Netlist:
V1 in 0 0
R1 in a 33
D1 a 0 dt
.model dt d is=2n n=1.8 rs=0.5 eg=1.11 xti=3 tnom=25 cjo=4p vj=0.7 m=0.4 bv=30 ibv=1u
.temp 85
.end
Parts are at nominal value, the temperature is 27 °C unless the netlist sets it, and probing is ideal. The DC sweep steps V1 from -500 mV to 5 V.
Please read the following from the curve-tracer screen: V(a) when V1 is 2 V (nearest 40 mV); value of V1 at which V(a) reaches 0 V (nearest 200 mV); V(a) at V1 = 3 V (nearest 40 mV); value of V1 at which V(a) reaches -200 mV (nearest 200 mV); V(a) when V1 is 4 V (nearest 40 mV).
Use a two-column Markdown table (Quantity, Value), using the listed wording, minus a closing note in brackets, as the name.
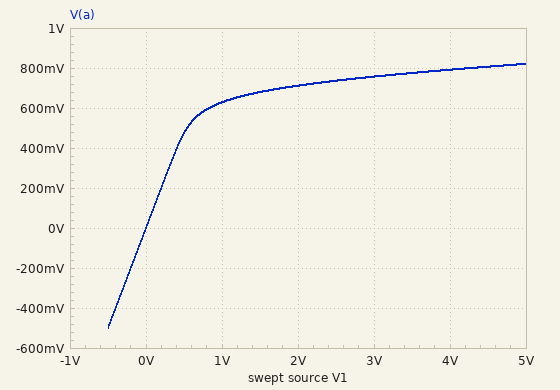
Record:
| Quantity | Value |
|---|---|
| V(a) when V1 is 2 V | 720 mV |
| value of V1 at which V(a) reaches 0 V | 0 V |
| V(a) at V1 = 3 V | 760 mV |
| value of V1 at which V(a) reaches -200 mV | -200 mV |
| V(a) when V1 is 4 V | 800 mV |
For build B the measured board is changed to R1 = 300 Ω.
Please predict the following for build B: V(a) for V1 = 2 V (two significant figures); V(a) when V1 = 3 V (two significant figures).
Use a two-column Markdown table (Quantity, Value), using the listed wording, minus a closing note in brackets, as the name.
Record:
| Quantity | Value |
|---|---|
| V(a) for V1 = 2 V | 580 mV |
| V(a) when V1 = 3 V | 610 mV |
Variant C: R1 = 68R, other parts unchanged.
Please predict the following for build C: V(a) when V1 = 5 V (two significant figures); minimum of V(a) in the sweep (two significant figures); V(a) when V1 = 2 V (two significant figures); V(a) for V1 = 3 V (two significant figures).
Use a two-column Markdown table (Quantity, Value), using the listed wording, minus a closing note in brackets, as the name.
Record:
| Quantity | Value |
|---|---|
| V(a) when V1 = 5 V | 750 mV |
| minimum of V(a) in the sweep | -500 mV |
| V(a) when V1 = 2 V | 660 mV |
| V(a) for V1 = 3 V | 700 mV |
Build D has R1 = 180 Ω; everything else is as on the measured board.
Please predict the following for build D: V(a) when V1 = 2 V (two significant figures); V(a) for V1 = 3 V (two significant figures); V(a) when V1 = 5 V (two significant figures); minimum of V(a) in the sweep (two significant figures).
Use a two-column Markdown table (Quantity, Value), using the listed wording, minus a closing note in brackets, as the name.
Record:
| Quantity | Value |
|---|---|
| V(a) when V1 = 2 V | 610 mV |
| V(a) for V1 = 3 V | 640 mV |
| V(a) when V1 = 5 V | 680 mV |
| minimum of V(a) in the sweep | -500 mV |
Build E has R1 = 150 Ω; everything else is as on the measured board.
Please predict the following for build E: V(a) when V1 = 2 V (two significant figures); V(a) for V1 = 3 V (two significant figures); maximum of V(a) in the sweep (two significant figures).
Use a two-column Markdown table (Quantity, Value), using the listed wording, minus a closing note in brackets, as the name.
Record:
| Quantity | Value |
|---|---|
| V(a) when V1 = 2 V | 620 mV |
| V(a) for V1 = 3 V | 650 mV |
| maximum of V(a) in the sweep | 690 mV |
